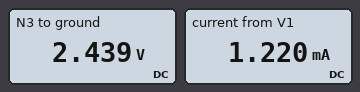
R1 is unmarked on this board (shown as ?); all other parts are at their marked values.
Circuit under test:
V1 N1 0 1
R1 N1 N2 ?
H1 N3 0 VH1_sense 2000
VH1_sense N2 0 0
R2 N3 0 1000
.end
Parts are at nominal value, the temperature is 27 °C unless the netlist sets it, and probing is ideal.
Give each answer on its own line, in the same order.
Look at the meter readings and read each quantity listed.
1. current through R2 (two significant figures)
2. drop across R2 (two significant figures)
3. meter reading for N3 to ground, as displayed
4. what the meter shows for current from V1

2.4 mA
2.4 V
2.439 V
1.220 mA
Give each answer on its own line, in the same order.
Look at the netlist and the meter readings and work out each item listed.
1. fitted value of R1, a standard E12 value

820 Ω
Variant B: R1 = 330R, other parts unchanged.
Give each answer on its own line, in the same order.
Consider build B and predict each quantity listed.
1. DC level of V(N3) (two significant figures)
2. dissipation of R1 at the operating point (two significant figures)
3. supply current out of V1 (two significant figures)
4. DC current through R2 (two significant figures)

6.1 V
3.0 mW
3.0 mA
6.1 mA
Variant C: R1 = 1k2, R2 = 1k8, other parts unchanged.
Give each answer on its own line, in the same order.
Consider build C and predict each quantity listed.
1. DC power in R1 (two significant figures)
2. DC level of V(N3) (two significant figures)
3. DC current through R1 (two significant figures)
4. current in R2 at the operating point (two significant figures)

830 µW
1.7 V
830 µA
930 µA
